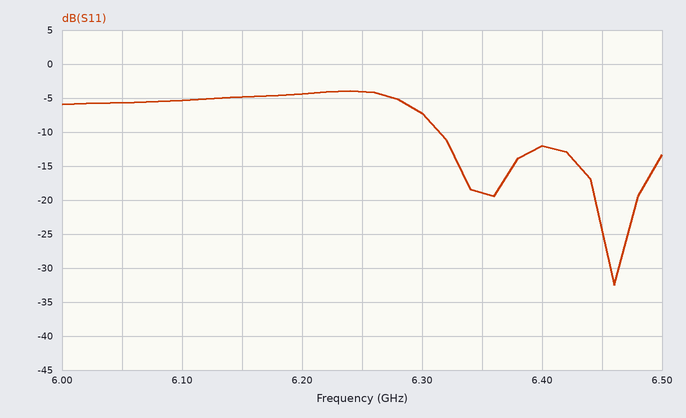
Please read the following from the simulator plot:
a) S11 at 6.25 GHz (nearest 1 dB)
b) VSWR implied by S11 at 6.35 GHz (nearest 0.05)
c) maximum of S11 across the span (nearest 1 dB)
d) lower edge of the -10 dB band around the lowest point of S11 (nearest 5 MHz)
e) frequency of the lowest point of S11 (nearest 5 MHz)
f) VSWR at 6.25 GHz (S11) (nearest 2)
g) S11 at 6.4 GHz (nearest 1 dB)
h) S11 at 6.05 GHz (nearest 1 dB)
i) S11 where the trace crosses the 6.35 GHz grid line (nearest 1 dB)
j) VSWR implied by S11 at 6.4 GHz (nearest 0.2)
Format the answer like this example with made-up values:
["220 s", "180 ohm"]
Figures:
["-4 dB", "1.25", "-4 dB", "6.315 GHz", "6.460 GHz", "4", "-12 dB", "-6 dB", "-19 dB", "1.6"]
